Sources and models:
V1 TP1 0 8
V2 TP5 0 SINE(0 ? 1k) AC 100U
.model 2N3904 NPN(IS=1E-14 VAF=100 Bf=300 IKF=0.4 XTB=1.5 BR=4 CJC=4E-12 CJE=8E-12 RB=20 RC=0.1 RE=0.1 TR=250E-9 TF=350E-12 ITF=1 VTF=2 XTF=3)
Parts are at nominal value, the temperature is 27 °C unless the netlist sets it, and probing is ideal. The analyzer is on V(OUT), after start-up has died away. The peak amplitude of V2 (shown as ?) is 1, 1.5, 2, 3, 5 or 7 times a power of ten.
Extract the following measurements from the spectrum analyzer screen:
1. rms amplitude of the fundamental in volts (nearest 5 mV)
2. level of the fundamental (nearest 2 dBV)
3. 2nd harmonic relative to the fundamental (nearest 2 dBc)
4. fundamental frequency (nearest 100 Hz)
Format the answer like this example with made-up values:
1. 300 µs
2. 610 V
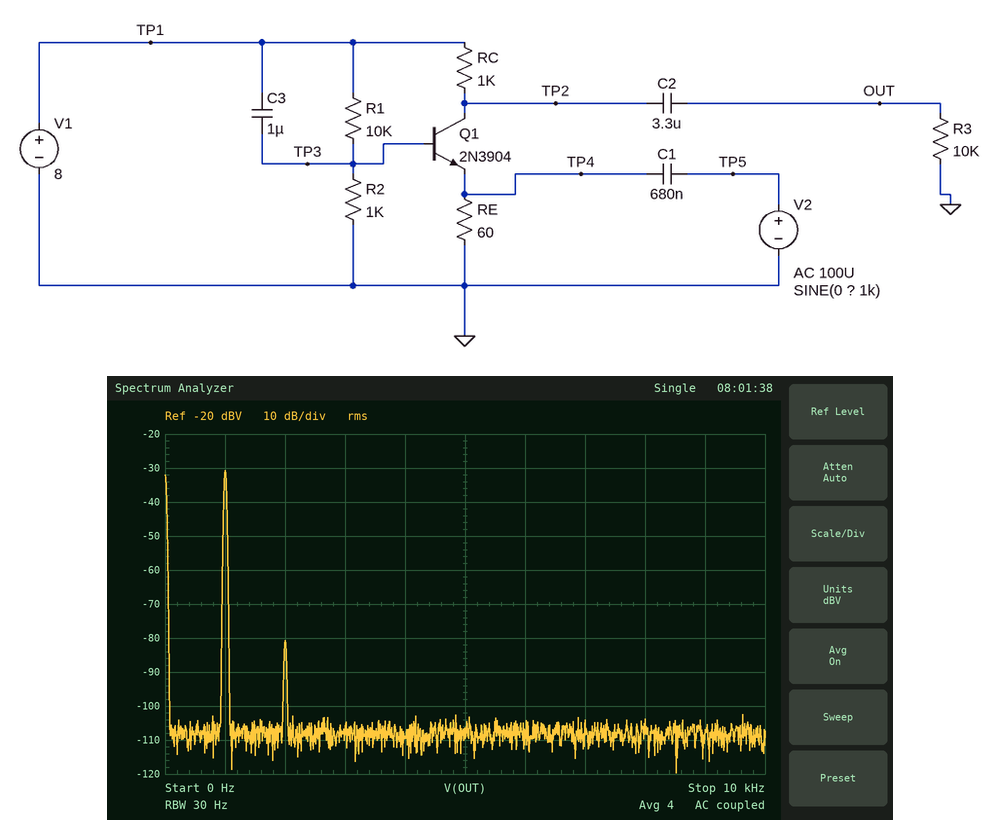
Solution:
1. 30 mV
2. -30 dBV
3. -50 dBc
4. 1.0 kHz
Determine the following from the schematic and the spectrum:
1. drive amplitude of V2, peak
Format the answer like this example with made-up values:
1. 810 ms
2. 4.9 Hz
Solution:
1. 15 mV
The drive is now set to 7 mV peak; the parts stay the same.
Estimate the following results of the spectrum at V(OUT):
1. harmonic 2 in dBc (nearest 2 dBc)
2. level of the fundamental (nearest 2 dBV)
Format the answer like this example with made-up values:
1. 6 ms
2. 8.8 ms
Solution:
1. -56 dBc
2. -38 dBV
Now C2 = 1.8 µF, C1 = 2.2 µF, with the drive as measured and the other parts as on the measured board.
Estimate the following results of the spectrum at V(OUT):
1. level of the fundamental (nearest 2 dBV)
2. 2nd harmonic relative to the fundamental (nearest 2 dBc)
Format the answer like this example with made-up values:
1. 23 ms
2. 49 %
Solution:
1. -20 dBV
2. -36 dBc
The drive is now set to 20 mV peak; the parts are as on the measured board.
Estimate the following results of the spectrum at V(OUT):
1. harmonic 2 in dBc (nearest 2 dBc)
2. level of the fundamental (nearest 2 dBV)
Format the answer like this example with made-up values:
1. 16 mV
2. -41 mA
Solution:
1. -48 dBc
2. -28 dBV
